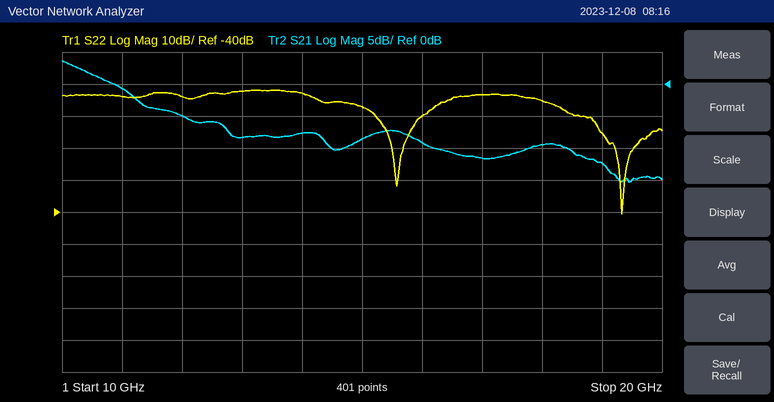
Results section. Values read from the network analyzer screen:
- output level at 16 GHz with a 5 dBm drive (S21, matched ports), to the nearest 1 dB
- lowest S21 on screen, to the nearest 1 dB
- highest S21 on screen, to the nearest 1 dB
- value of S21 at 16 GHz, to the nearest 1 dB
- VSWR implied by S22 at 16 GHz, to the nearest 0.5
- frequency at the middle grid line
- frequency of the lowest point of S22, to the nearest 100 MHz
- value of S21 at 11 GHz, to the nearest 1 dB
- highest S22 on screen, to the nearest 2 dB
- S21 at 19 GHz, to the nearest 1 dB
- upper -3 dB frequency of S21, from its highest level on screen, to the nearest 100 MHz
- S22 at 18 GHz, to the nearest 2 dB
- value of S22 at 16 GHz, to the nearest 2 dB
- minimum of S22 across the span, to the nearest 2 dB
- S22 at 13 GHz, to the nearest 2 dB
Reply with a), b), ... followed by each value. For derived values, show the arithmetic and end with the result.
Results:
a) 5 dBm + (-9 dB) = -4 dBm
b) -15 dB
c) 4 dB
d) -9 dB
e) |Γ| = 10^(-10/20) = 0.3162; VSWR = (1 + 0.3162)/(1 − 0.3162) ≈ 1.92, so 2.0 to the nearest 0.5
f) 15 GHz
g) 19.3 GHz
h) -1 dB
i) -2 dB
j) -12 dB
k) 10.7 GHz
l) -6 dB
m) -10 dB
n) -40 dB
o) -2 dB
